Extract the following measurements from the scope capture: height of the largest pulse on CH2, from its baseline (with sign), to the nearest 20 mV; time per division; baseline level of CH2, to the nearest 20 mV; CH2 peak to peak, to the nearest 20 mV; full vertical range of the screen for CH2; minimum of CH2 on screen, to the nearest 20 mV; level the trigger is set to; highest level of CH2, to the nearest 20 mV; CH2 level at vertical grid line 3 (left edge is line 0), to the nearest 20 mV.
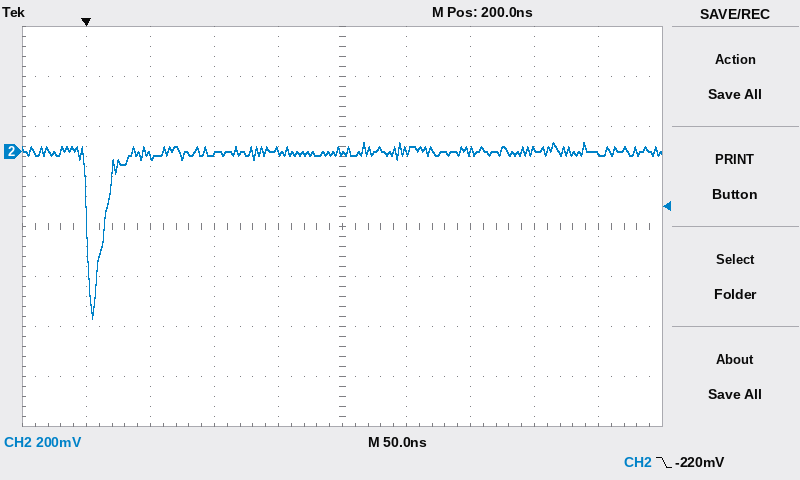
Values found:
-660 mV
50 ns
0 mV
700 mV
1.6 V
-660 mV
-220 mV
40 mV
0 mV
